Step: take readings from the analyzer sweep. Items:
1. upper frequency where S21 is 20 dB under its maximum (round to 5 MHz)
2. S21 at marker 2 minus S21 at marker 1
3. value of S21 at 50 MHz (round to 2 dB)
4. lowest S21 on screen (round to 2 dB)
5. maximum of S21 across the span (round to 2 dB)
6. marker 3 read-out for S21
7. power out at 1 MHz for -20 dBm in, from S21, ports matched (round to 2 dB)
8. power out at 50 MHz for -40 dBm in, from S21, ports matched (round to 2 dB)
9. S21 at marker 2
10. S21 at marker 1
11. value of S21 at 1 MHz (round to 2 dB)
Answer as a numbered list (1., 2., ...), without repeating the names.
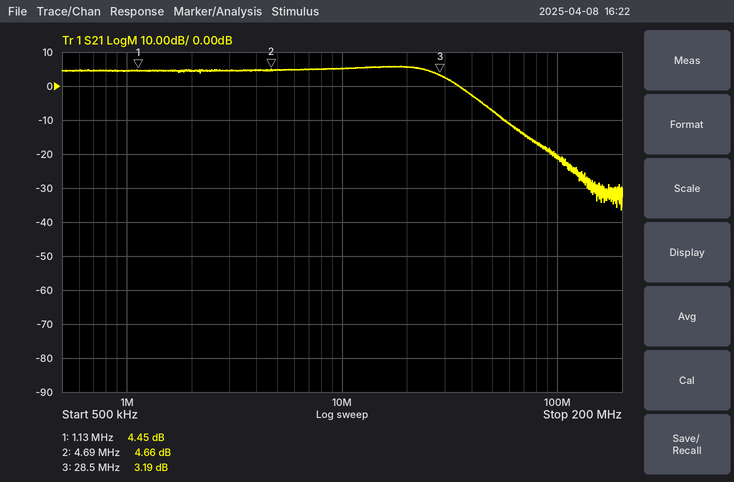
1. 70 MHz
2. 0.21 dB
3. -8 dB
4. -36 dB
5. 6 dB
6. 3.19 dB
7. -16 dBm
8. -48 dBm
9. 4.66 dB
10. 4.45 dB
11. 4 dB
